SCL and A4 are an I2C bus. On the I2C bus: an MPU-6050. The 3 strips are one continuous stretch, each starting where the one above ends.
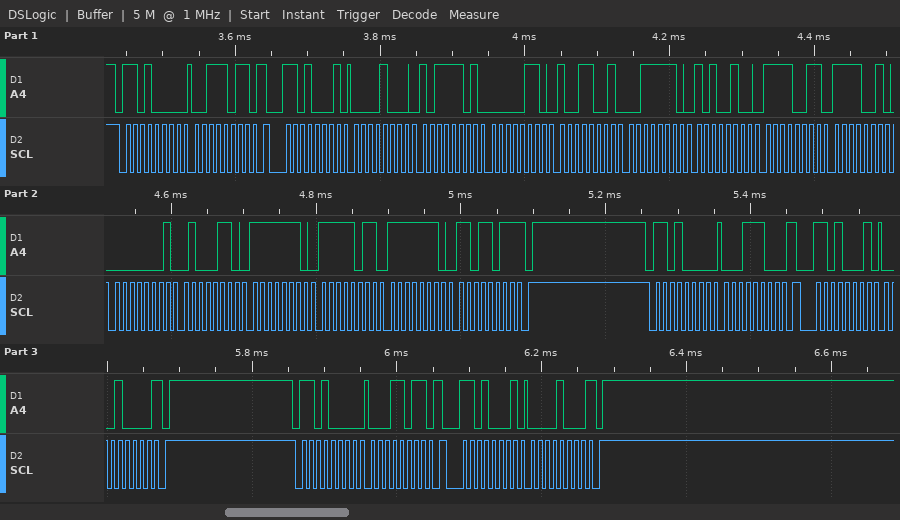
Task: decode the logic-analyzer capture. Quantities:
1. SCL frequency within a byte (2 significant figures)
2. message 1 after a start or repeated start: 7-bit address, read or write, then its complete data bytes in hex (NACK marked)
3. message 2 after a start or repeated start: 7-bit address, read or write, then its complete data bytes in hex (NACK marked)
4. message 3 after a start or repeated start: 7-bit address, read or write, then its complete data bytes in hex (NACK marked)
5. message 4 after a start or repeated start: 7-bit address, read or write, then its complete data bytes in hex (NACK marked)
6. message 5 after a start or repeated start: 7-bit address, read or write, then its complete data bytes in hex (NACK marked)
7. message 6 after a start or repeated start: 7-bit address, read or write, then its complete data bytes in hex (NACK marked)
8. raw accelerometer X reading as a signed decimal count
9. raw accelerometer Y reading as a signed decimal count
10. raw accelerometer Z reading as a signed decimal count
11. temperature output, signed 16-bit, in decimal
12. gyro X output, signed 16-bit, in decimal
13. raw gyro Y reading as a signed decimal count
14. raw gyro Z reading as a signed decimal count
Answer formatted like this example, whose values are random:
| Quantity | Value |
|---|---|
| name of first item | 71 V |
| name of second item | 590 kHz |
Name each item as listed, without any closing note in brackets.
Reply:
| Quantity | Value |
|---|---|
| SCL frequency within a byte | 100 kHz |
| message 1 after a start or repeated start: 7-bit address, read or write, then its complete data bytes in hex | 0x68 write: 3B |
| message 2 after a start or repeated start: 7-bit address, read or write, then its complete data bytes in hex | 0x68 read: 08 BD 06 99 3E A4 F3 F2 01 46 FE FB FE DB NACK |
| message 3 after a start or repeated start: 7-bit address, read or write, then its complete data bytes in hex | 0x68 write: 1C |
| message 4 after a start or repeated start: 7-bit address, read or write, then its complete data bytes in hex | 0x68 read: 10 NACK |
| message 5 after a start or repeated start: 7-bit address, read or write, then its complete data bytes in hex | 0x68 write: 1B |
| message 6 after a start or repeated start: 7-bit address, read or write, then its complete data bytes in hex | 0x68 read: 08 NACK |
| raw accelerometer X reading as a signed decimal count | 2237 |
| raw accelerometer Y reading as a signed decimal count | 1689 |
| raw accelerometer Z reading as a signed decimal count | 16036 |
| temperature output, signed 16-bit, in decimal | -3086 |
| gyro X output, signed 16-bit, in decimal | 326 |
| raw gyro Y reading as a signed decimal count | -261 |
| raw gyro Z reading as a signed decimal count | -293 |
